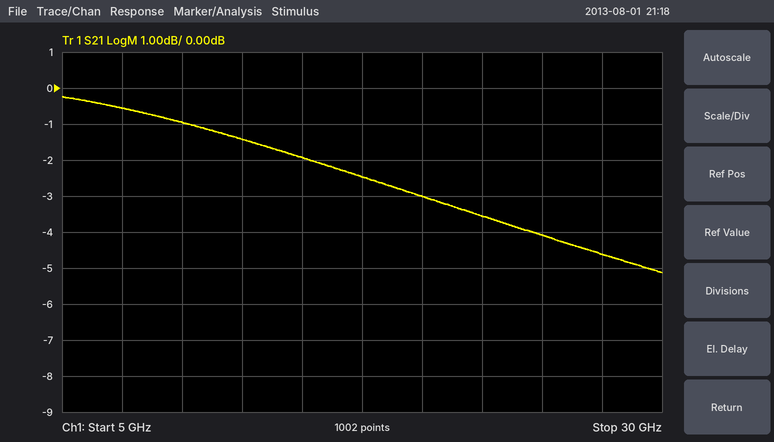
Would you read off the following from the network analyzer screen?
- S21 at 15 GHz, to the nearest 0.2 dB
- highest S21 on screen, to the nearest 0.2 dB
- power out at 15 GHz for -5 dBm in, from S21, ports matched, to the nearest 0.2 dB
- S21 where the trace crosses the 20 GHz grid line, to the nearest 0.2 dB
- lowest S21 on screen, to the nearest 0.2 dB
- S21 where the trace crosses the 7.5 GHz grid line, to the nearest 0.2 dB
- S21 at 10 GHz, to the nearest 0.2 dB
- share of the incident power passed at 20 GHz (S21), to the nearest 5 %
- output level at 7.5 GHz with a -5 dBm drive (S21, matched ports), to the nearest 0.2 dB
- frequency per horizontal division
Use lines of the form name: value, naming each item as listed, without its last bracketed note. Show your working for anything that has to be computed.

S21 at 15 GHz, to the nearest 0.2 dB: -2.0 dB
highest S21 on screen, to the nearest 0.2 dB: -0.2 dB
power out at 15 GHz for -5 dBm in, from S21, ports matched, to the nearest 0.2 dB: -5 dBm + (-2.0 dB) = -7.0 dBm
S21 where the trace crosses the 20 GHz grid line, to the nearest 0.2 dB: -3.0 dB
lowest S21 on screen, to the nearest 0.2 dB: -5.2 dB
S21 where the trace crosses the 7.5 GHz grid line, to the nearest 0.2 dB: -0.6 dB
S21 at 10 GHz, to the nearest 0.2 dB: -1.0 dB
share of the incident power passed at 20 GHz (S21), to the nearest 5 %: 10^(-3/10) ≈ 50 %
output level at 7.5 GHz with a -5 dBm drive (S21, matched ports), to the nearest 0.2 dB: -5 dBm + (-0.6 dB) = -5.6 dBm
frequency per horizontal division: 2.5 GHz
